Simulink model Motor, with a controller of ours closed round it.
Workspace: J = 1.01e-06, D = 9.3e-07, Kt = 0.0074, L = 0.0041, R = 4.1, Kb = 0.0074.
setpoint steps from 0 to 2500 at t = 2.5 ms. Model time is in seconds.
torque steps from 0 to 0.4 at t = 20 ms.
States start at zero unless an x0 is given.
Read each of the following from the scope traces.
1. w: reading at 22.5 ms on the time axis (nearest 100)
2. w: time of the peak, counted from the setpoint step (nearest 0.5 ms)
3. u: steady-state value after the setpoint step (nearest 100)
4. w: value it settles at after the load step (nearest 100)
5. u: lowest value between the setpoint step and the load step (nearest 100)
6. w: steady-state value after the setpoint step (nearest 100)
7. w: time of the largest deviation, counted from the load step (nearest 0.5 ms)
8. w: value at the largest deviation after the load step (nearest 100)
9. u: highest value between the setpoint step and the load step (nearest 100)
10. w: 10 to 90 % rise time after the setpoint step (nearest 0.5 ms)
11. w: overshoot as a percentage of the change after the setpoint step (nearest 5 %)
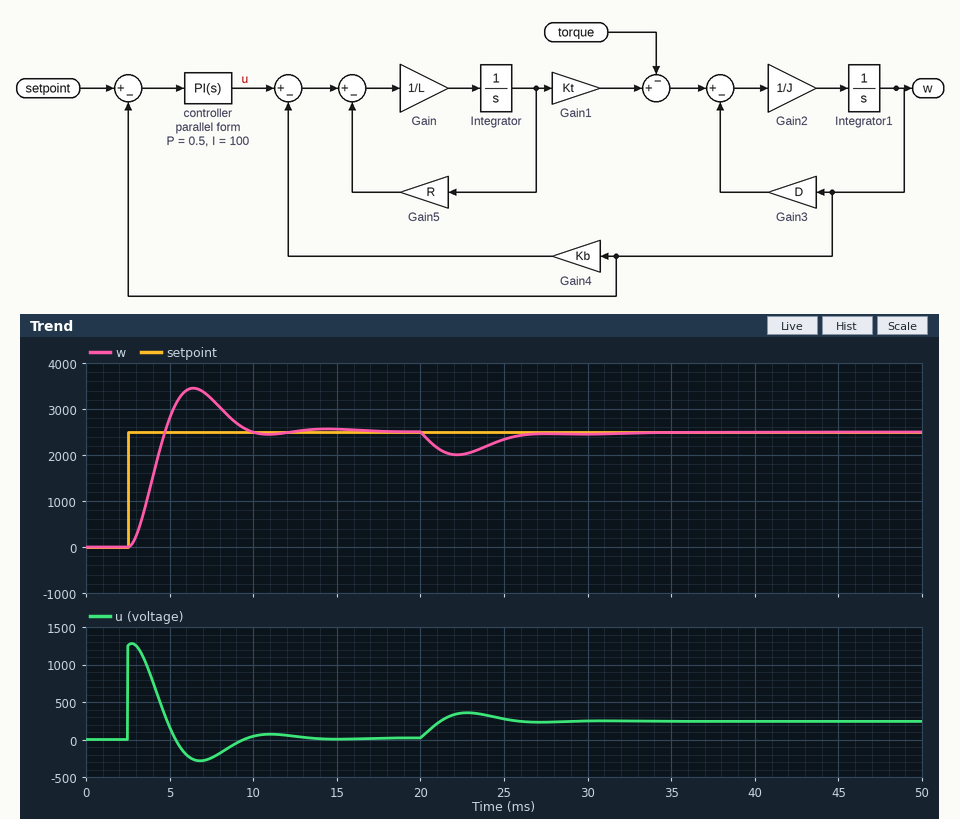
2000
4.0 ms
0
2500
-300
2500
2.0 ms
2000
1300
1.5 ms
40 %
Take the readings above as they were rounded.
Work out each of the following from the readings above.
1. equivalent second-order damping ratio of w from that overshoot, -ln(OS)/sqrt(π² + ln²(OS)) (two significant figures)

0.28
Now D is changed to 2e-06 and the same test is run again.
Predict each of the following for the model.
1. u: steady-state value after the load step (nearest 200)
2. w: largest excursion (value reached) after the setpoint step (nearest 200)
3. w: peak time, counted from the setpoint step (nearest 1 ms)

200
3400
4 ms
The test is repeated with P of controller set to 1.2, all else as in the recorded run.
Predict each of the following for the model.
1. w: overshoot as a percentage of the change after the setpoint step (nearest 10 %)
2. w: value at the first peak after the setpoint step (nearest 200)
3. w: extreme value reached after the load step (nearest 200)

40 %
3400
2200
